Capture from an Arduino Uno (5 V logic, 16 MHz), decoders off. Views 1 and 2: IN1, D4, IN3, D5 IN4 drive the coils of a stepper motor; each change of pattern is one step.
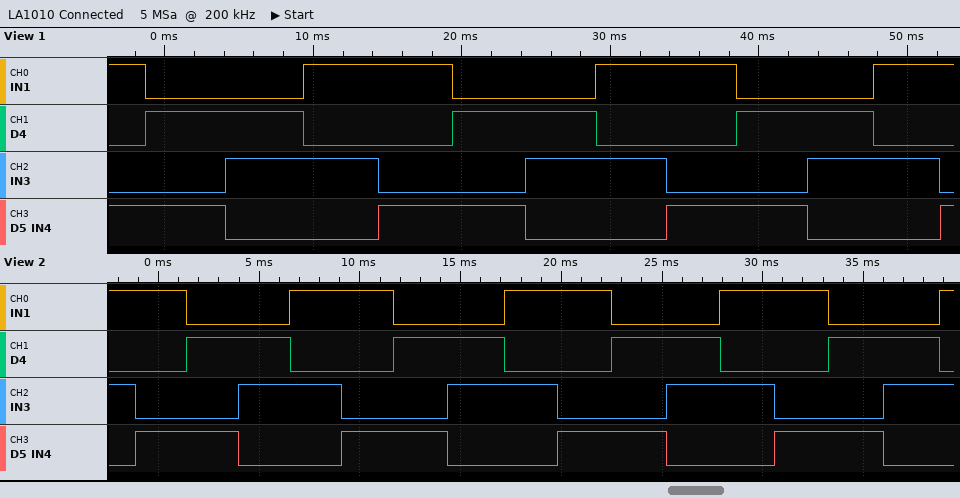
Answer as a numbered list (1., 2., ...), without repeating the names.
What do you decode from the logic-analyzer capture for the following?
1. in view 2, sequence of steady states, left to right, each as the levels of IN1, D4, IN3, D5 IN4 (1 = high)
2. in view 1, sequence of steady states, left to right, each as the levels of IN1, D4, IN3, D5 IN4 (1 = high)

1. 1010 1001 0101 0110 1010 1001 0101 0110 1010 1001 0101 0110 1010 1001 0101 0110 1010
2. 1001 0101 0110 1010 1001 0101 0110 1010 1001 0101 0110 1010 1001
